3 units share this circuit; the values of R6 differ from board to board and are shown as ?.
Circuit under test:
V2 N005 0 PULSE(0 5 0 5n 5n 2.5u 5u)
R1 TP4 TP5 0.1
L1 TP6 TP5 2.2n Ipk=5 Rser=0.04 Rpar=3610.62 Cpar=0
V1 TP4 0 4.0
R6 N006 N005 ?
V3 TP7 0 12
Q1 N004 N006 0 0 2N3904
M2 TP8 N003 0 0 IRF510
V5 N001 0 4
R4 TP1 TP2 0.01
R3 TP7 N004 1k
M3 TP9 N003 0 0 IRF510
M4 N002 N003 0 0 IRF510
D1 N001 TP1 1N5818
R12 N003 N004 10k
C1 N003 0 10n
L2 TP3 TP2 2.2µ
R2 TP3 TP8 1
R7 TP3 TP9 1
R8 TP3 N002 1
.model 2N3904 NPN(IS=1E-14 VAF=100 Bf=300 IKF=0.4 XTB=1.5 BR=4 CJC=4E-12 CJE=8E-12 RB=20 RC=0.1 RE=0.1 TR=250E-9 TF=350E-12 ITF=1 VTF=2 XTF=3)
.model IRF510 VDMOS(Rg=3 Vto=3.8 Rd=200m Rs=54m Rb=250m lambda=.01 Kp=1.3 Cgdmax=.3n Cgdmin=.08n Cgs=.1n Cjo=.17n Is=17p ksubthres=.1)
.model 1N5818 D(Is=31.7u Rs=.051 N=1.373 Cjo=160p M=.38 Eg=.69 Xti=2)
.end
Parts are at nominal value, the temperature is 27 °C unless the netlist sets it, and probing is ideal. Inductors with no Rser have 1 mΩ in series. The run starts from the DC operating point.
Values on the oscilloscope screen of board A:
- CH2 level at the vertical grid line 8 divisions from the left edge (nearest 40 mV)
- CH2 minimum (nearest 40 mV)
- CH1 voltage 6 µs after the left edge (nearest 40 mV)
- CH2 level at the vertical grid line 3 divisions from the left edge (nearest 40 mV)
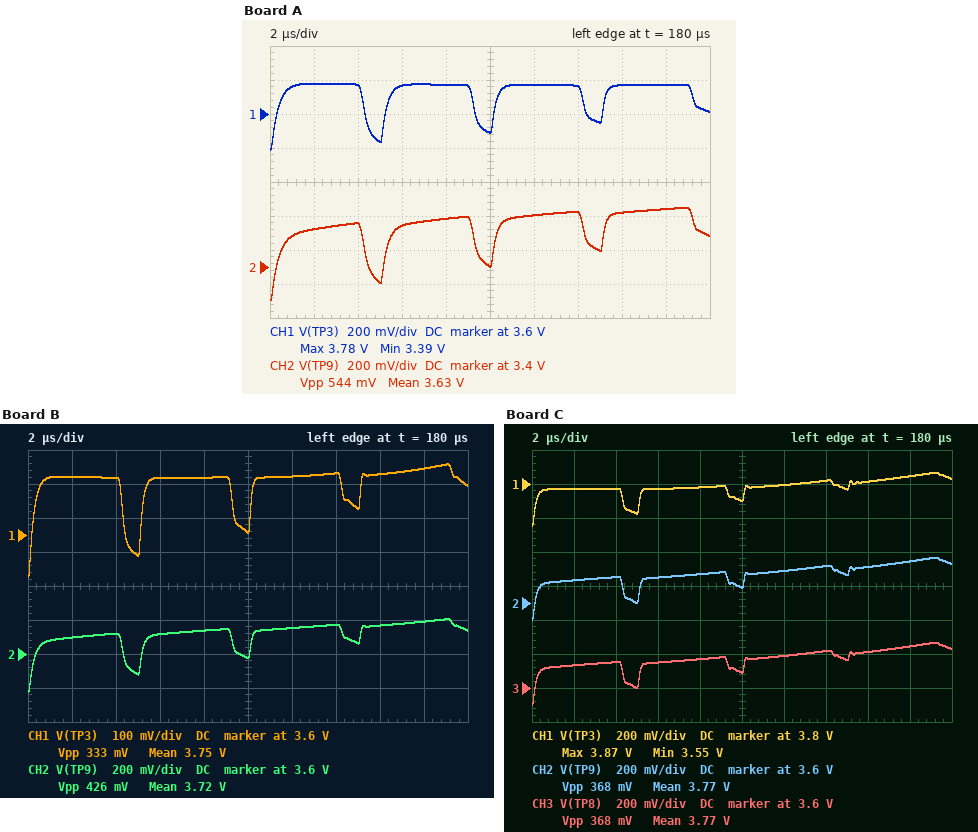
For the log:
3.72 V
3.20 V
3.76 V
3.64 V
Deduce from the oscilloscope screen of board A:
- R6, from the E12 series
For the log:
8.2 kΩ
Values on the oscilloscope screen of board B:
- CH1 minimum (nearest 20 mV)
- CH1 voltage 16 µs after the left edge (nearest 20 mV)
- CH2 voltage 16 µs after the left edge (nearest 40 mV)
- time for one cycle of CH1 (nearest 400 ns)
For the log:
3.48 V
3.78 V
3.76 V
4.8 µs
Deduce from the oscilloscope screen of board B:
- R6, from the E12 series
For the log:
5.6 kΩ
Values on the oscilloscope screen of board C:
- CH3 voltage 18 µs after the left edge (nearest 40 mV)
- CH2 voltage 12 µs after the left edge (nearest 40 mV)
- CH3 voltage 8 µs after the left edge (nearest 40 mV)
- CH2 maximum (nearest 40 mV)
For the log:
3.84 V
3.80 V
3.76 V
3.88 V
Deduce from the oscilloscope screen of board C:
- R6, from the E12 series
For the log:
3.9 kΩ
